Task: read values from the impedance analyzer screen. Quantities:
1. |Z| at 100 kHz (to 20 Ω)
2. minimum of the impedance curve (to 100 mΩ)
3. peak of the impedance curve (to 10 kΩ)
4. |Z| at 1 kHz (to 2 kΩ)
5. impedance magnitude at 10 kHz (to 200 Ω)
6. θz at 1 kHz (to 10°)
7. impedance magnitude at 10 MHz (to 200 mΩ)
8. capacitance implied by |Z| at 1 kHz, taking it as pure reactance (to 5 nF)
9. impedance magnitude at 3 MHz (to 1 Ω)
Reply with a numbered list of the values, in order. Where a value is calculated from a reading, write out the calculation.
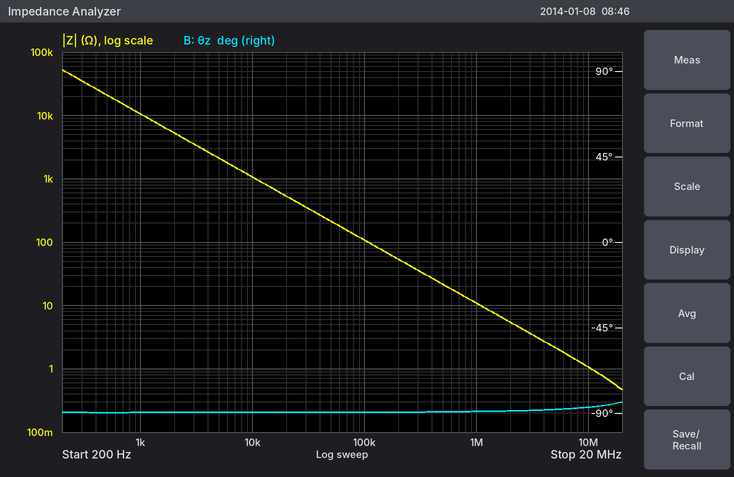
1. 100 Ω
2. 500 mΩ
3. 50 kΩ
4. 10 kΩ
5. 1.0 kΩ
6. -90°
7. 1.0 Ω
8. C = 1/(2π × 1 kHz × 10 kΩ) ≈ 15.9 nF, so 15 nF to the nearest 5 nF
9. 4 Ω
